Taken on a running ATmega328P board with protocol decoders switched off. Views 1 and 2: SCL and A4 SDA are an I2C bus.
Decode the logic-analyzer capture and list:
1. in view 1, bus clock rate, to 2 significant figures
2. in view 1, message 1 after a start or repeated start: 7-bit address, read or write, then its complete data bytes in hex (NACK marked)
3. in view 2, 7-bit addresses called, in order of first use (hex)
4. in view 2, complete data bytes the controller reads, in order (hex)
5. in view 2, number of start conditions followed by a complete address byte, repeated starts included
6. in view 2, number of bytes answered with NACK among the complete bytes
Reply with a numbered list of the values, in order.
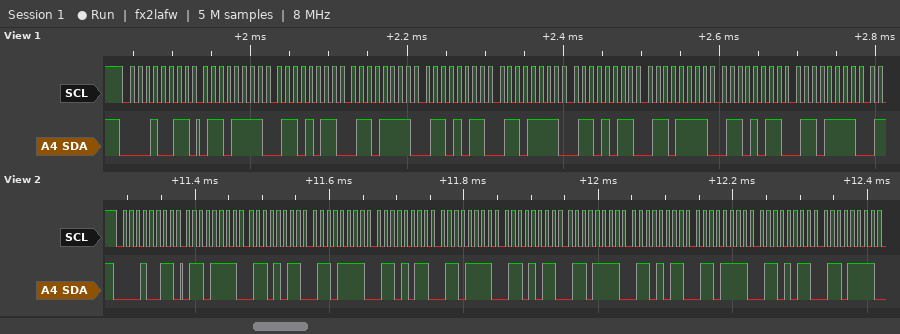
1. 100 kHz
2. 0x09 read: 6F 6B 6F 6B 6F 6B 6F 6B 6F
3. 0x09
4. 6F 6B 6F 6B 6F 6B 6F 6B 6F 6B 6F
5. 1
6. 0
